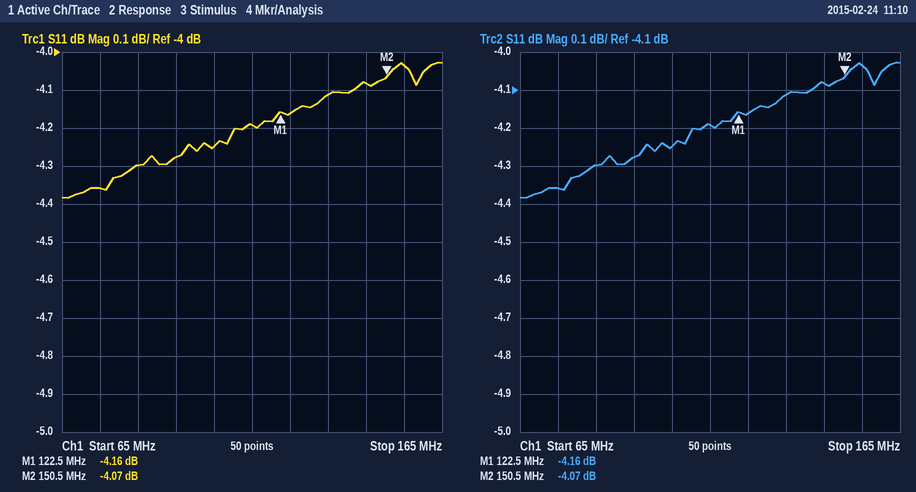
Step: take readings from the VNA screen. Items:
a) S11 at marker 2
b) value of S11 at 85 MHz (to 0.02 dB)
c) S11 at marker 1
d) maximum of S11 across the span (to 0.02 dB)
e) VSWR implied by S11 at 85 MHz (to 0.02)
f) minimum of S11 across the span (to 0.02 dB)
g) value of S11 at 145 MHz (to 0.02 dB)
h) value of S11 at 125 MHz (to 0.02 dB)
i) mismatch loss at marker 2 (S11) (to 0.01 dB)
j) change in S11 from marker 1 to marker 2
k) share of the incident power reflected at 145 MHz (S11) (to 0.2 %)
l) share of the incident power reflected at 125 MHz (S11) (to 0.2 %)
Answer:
-4.07 dB
-4.30 dB
-4.16 dB
-4.02 dB
4.12
-4.38 dB
-4.08 dB
-4.16 dB
2.16 dB
0.09 dB
39.0 %
38.4 %
